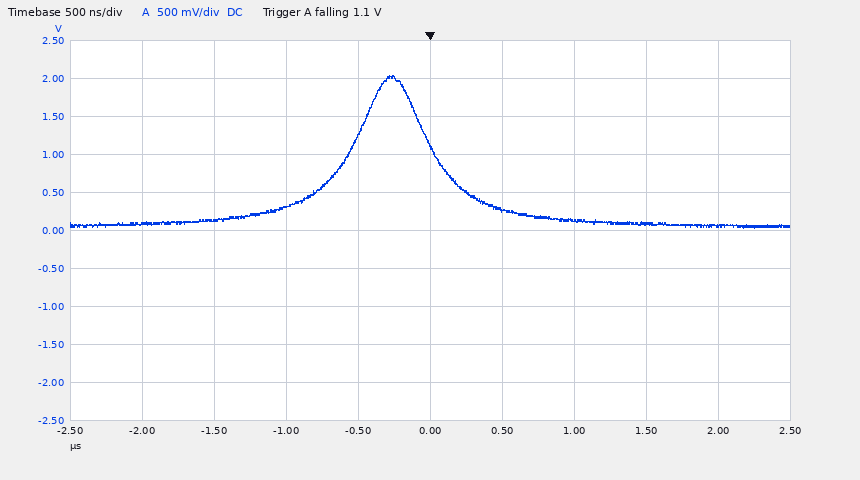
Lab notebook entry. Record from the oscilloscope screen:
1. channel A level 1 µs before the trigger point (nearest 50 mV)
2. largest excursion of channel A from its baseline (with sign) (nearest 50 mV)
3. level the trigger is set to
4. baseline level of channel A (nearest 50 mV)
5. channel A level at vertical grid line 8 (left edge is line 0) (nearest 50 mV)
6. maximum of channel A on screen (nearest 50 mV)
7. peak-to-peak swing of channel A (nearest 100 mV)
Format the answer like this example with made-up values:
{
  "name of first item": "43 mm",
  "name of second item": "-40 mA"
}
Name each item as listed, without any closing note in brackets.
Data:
{
  "channel A level 1 µs before the trigger point": "300 mV",
  "largest excursion of channel A from its baseline (with sign)": "+1.95 V",
  "level the trigger is set to": "1.1 V",
  "baseline level of channel A": "100 mV",
  "channel A level at vertical grid line 8 (left edge is line 0)": "100 mV",
  "maximum of channel A on screen": "2.05 V",
  "peak-to-peak swing of channel A": "2.00 V"
}
